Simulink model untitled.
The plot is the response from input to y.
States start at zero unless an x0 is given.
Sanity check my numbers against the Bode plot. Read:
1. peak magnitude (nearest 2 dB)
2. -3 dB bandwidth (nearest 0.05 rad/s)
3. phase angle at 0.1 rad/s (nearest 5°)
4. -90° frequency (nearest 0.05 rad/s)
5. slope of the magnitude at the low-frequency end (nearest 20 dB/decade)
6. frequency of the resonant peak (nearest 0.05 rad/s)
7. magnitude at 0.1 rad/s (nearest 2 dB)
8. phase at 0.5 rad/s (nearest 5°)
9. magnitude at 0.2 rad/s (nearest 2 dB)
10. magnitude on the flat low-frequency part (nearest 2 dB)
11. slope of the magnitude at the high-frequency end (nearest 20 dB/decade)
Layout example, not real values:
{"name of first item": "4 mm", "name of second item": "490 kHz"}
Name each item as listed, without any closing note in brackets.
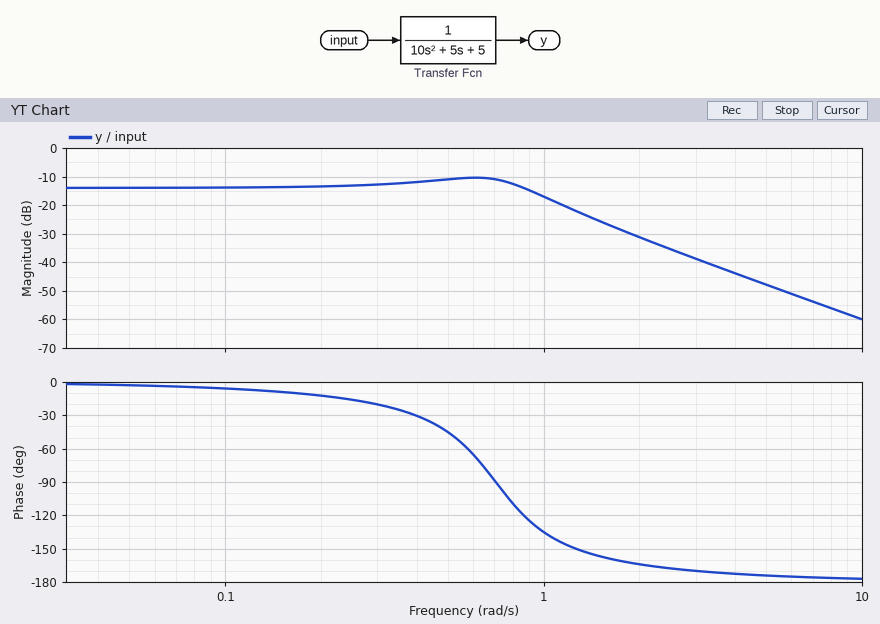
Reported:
{"peak magnitude": "-10 dB", "-3 dB bandwidth": "1.00 rad/s", "phase angle at 0.1 rad/s": "-5°", "-90° frequency": "0.70 rad/s", "slope of the magnitude at the low-frequency end": "0 dB/decade", "frequency of the resonant peak": "0.60 rad/s", "magnitude at 0.1 rad/s": "-14 dB", "phase at 0.5 rad/s": "-45°", "magnitude at 0.2 rad/s": "-14 dB", "magnitude on the flat low-frequency part": "-14 dB", "slope of the magnitude at the high-frequency end": "-40 dB/decade"}
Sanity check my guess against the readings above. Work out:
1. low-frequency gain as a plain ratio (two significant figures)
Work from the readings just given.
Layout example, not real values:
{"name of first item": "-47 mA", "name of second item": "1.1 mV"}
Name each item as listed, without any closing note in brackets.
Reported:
{"low-frequency gain as a plain ratio": "0.20"}
